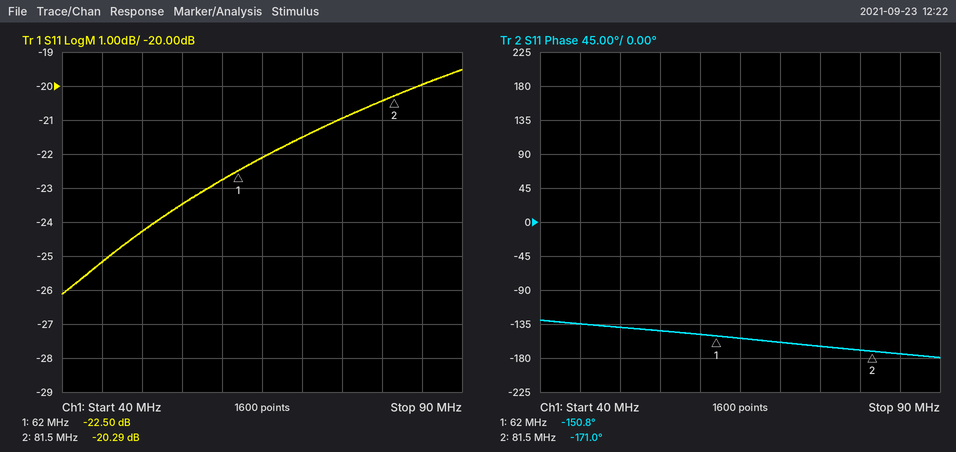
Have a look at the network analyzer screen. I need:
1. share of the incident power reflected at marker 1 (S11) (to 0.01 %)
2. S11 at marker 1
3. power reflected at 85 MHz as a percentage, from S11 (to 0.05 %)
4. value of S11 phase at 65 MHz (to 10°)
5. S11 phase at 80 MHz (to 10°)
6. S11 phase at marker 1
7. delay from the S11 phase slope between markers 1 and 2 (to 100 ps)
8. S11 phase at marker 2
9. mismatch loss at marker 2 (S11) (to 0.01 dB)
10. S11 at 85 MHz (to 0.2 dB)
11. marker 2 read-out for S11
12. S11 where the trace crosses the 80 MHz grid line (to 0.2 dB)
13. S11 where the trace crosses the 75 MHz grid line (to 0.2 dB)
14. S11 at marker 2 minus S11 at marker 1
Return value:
0.56 %
-22.50 dB
1.00 %
-150°
-170°
-150.8°
2.9 ns
-171.0°
0.04 dB
-20.0 dB
-20.29 dB
-20.4 dB
-21.0 dB
2.21 dB
